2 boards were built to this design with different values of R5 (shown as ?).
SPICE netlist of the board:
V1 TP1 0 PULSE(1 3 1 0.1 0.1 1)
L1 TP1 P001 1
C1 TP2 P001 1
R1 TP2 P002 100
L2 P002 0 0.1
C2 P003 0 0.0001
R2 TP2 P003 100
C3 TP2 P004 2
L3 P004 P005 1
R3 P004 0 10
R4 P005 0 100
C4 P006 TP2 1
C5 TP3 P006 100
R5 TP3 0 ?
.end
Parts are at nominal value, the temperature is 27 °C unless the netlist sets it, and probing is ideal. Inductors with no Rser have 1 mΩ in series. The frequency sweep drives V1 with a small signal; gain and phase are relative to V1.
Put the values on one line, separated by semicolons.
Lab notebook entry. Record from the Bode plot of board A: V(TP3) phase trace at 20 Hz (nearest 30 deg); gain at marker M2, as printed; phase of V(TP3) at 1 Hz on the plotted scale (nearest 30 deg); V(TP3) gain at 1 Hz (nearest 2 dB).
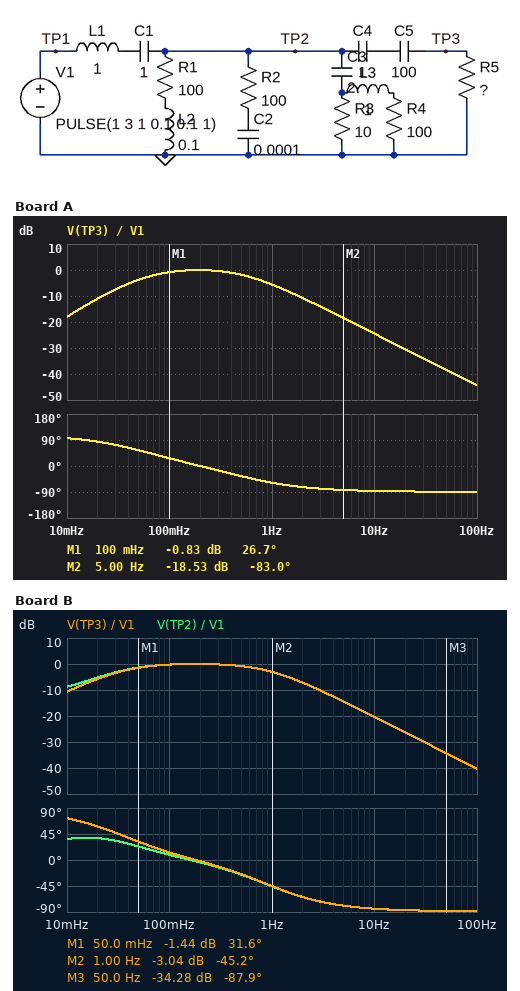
-90 deg; -18.53 dB; -60 deg; -6 dB
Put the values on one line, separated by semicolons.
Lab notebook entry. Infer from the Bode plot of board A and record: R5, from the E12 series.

6.8 Ω
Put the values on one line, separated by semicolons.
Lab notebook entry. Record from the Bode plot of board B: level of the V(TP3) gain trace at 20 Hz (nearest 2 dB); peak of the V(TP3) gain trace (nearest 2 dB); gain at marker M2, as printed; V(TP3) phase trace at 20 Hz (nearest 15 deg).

-26 dB; 0 dB; -3.04 dB; -90 deg
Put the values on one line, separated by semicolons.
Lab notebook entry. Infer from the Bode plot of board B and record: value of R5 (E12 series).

22 Ω
